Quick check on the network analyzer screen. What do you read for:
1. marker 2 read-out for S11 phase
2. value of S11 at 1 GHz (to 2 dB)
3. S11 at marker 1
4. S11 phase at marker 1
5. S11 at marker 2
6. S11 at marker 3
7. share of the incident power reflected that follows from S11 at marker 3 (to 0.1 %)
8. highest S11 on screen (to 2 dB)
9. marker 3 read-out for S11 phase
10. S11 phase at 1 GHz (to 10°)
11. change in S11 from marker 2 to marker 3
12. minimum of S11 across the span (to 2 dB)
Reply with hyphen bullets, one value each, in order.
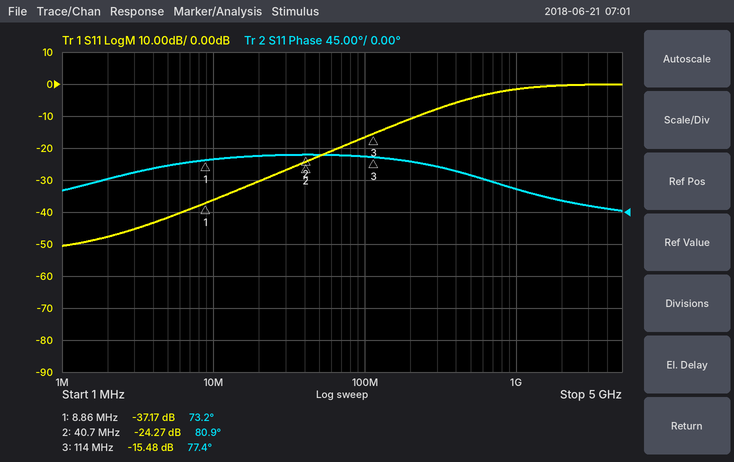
- 80.9°
- -2 dB
- -37.17 dB
- 73.2°
- -24.27 dB
- -15.48 dB
- 2.8 %
- 0 dB
- 77.4°
- 30°
- 8.79 dB
- -50 dB
